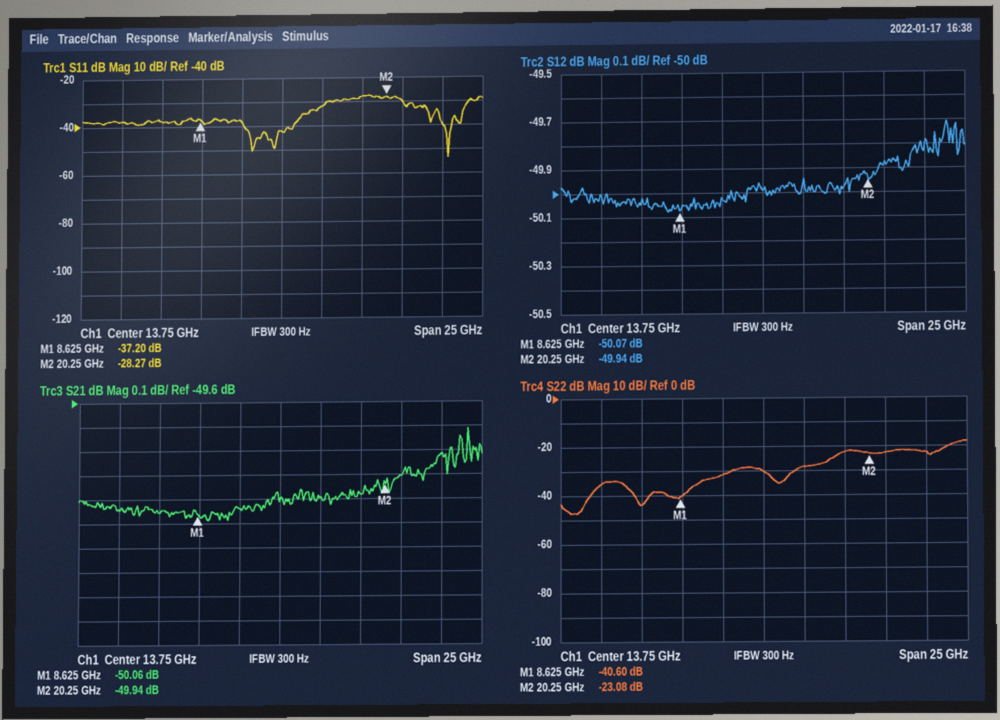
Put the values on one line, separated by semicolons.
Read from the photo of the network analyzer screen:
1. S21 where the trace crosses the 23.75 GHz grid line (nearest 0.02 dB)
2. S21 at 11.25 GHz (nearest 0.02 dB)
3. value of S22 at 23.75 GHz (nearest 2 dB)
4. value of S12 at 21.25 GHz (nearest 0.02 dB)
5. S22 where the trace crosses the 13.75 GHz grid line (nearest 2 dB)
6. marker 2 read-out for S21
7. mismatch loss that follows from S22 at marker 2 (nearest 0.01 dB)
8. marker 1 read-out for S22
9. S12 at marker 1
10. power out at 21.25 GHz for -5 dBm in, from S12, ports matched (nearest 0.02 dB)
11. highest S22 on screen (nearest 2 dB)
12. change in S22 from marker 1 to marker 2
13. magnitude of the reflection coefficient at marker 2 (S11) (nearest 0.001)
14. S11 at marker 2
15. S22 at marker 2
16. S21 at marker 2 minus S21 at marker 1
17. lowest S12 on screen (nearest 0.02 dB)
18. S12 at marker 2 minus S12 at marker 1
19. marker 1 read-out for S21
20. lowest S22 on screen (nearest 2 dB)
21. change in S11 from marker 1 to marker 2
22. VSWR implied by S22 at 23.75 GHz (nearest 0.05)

-49.82 dB; -50.04 dB; -22 dB; -49.88 dB; -30 dB; -49.94 dB; 0.02 dB; -40.60 dB; -50.07 dB; -54.88 dBm; -18 dB; 17.52 dB; 0.039; -28.27 dB; -23.08 dB; 0.12 dB; -50.08 dB; 0.13 dB; -50.06 dB; -48 dB; 8.93 dB; 1.15
